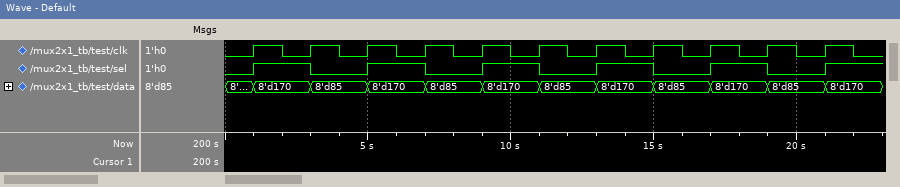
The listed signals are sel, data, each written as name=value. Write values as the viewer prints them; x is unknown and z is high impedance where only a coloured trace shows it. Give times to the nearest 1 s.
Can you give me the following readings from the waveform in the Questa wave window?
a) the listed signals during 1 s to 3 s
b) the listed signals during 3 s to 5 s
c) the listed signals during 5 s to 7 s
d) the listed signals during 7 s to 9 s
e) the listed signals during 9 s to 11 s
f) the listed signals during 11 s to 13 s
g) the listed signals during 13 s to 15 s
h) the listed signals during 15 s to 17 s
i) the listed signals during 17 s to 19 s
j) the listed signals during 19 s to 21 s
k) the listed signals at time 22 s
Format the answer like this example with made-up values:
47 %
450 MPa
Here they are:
sel=1, data=8'd170
sel=0, data=8'd85
sel=1, data=8'd170
sel=0, data=8'd85
sel=1, data=8'd170
sel=0, data=8'd85
sel=1, data=8'd170
sel=0, data=8'd85
sel=1, data=8'd170
sel=0, data=8'd85
sel=1, data=8'd170
